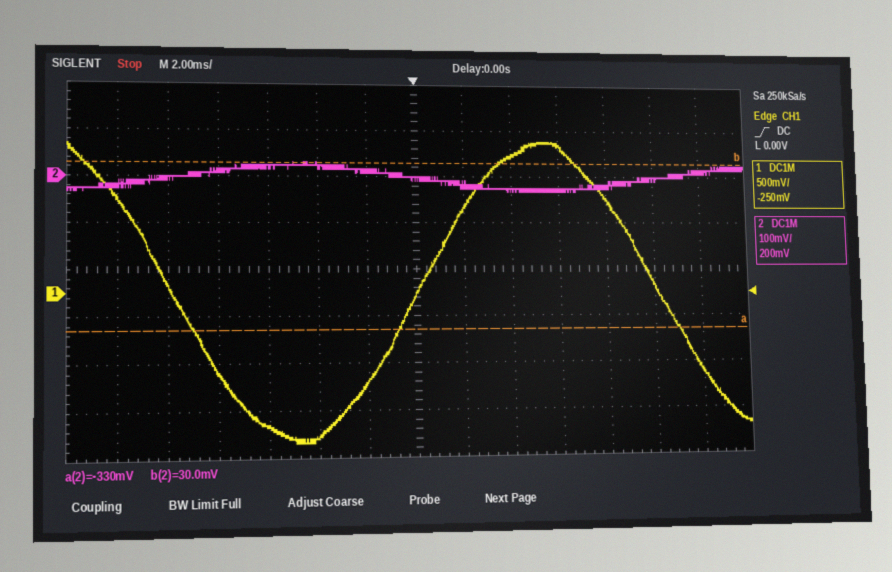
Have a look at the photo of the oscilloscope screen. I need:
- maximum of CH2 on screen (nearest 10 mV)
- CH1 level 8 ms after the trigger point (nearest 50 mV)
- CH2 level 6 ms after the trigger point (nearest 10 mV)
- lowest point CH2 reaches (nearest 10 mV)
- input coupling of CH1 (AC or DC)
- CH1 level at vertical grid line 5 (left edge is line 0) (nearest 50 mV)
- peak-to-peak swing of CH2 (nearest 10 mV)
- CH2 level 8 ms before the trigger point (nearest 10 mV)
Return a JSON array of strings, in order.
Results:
["30 mV", "1.00 V", "-30 mV", "-30 mV", "DC", "-1.50 V", "60 mV", "10 mV"]
